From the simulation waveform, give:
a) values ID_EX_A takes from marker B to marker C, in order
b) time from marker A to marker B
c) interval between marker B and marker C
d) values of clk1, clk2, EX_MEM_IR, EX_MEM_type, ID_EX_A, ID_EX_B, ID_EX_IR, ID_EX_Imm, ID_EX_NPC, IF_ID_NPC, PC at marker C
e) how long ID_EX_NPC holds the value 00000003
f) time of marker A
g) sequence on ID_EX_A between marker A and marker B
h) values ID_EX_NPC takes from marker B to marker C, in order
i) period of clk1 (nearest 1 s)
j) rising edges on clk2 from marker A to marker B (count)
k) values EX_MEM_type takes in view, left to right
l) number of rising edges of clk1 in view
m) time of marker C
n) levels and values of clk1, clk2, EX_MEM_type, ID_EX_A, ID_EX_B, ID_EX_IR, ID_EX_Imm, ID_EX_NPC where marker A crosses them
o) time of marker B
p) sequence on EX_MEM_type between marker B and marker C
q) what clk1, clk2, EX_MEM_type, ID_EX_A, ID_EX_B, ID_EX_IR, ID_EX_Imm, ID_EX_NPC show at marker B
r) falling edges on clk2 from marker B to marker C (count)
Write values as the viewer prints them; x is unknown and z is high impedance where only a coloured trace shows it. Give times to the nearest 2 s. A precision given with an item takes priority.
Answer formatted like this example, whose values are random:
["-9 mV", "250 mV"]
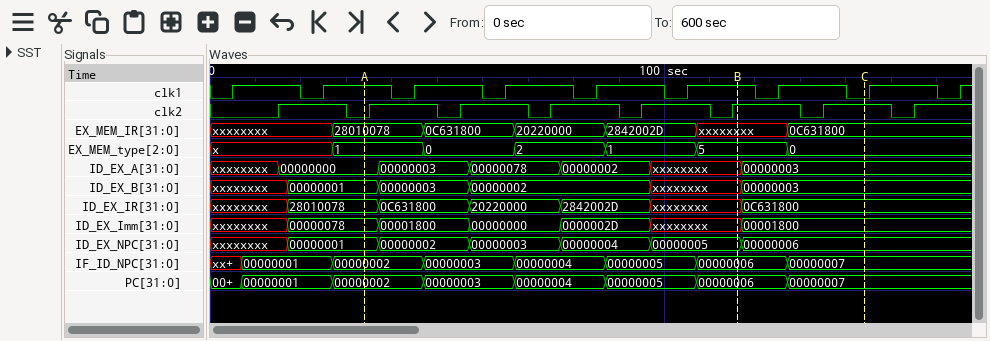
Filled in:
["xxxxxxxx, 00000003", "82 s", "28 s", "clk1=0, clk2=1, EX_MEM_IR=0C631800, EX_MEM_type=0, ID_EX_A=00000003, ID_EX_B=00000003, ID_EX_IR=0C631800, ID_EX_Imm=00001800, ID_EX_NPC=00000006, IF_ID_NPC=00000007, PC=00000007", "20 s", "34 s", "00000000, 00000003, 00000078, 00000002, xxxxxxxx", "00000005, 00000006", "20 s", "5", "x, 1, 0, 2, 1, 5, 0", "9", "144 s", "clk1=1, clk2=0, EX_MEM_type=1, ID_EX_A=00000000, ID_EX_B=00000001, ID_EX_IR=28010078, ID_EX_Imm=00000078, ID_EX_NPC=00000001", "116 s", "5, 0", "clk1=1, clk2=1, EX_MEM_type=5, ID_EX_A=xxxxxxxx, ID_EX_B=xxxxxxxx, ID_EX_IR=xxxxxxxx, ID_EX_Imm=xxxxxxxx, ID_EX_NPC=00000005", "1"]
